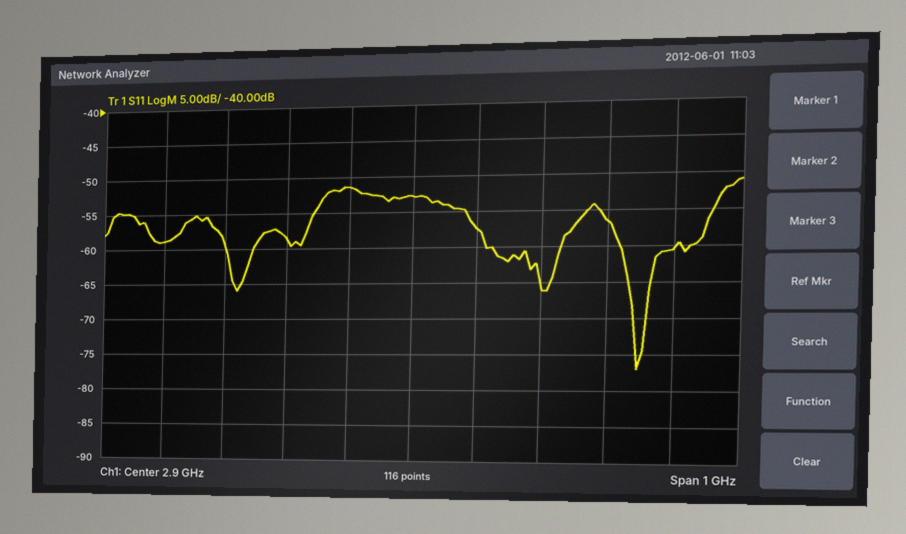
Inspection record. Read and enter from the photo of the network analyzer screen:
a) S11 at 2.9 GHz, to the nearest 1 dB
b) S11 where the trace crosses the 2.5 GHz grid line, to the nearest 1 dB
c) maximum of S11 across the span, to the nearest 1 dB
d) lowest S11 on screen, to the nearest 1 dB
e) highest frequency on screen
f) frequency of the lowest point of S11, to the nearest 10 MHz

-53 dB
-59 dB
-51 dB
-77 dB
3.4 GHz
3.25 GHz
